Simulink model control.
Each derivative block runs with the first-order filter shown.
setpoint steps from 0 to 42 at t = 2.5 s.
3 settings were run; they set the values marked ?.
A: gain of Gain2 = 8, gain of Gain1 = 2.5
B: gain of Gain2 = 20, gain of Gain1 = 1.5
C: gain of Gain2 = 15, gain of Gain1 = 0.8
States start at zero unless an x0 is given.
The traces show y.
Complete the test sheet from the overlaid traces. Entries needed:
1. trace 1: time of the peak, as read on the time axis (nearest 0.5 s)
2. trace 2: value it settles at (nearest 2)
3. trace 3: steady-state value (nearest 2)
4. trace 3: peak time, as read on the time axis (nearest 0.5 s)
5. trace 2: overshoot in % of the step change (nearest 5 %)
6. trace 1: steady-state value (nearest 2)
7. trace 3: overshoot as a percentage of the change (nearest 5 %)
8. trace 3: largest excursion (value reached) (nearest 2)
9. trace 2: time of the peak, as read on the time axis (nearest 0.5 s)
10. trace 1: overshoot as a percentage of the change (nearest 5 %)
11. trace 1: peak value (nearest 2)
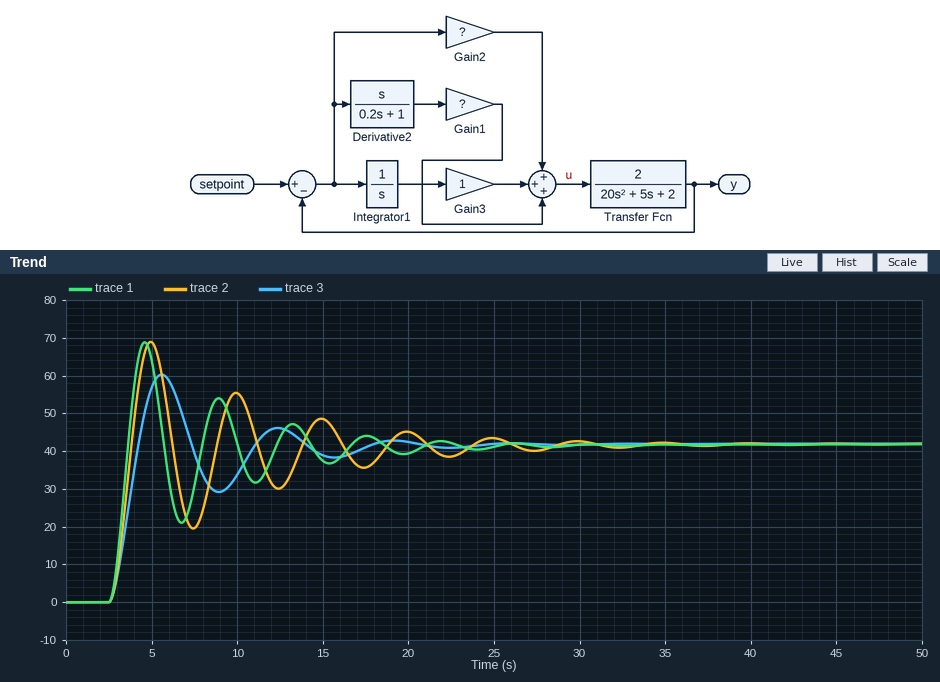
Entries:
4.5 s
42
42
5.5 s
65 %
42
45 %
60
5.0 s
65 %
68
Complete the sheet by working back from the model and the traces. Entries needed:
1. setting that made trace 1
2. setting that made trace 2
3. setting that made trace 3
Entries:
B
C
A
